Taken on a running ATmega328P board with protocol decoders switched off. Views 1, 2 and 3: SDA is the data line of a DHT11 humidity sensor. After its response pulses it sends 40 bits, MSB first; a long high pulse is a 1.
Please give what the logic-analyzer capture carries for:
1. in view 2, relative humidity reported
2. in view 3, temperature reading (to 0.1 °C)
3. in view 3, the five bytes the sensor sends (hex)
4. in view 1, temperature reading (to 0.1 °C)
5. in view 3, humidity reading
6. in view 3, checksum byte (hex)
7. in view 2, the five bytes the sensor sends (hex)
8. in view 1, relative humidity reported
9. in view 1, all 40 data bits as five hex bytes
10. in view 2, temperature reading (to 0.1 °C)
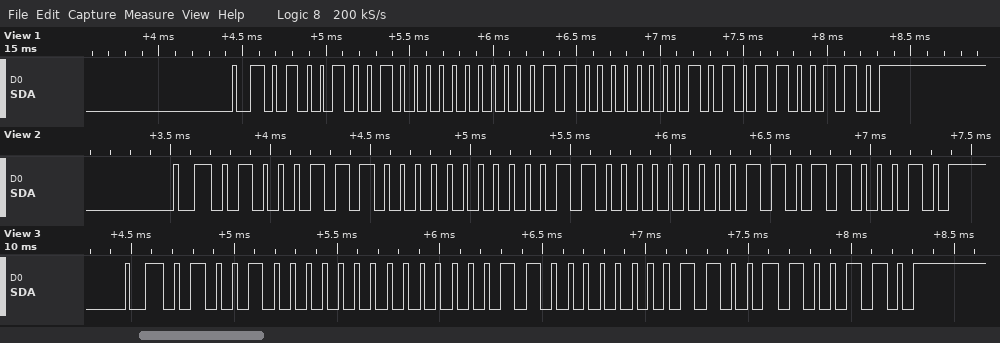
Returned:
71 %
24.6 °C
48 00 18 06 66
24.5 °C
72 %
0x66
47 00 18 03 62
73 %
49 00 18 05 66
24.3 °C
